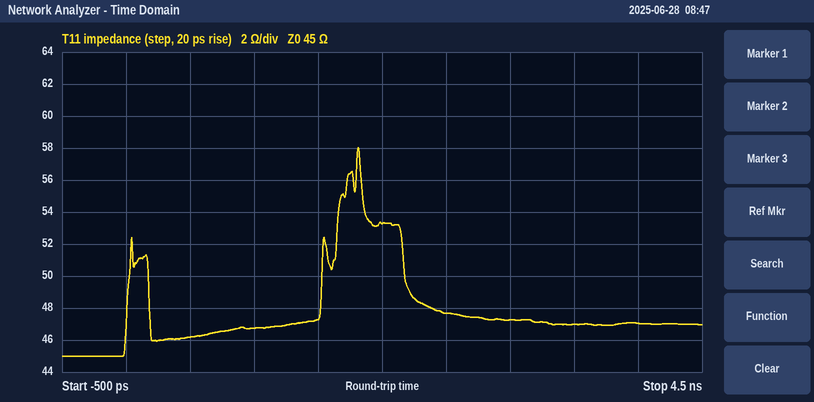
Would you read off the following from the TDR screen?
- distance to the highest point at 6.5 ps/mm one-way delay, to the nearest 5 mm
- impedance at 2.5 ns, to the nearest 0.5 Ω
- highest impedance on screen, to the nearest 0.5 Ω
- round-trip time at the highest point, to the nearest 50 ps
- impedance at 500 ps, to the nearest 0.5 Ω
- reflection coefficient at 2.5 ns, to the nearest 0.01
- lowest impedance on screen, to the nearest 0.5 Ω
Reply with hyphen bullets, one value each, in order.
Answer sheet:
- 140 mm
- 47.5 Ω
- 58.0 Ω
- 1.80 ns
- 46.0 Ω
- +0.03
- 45.0 Ω
